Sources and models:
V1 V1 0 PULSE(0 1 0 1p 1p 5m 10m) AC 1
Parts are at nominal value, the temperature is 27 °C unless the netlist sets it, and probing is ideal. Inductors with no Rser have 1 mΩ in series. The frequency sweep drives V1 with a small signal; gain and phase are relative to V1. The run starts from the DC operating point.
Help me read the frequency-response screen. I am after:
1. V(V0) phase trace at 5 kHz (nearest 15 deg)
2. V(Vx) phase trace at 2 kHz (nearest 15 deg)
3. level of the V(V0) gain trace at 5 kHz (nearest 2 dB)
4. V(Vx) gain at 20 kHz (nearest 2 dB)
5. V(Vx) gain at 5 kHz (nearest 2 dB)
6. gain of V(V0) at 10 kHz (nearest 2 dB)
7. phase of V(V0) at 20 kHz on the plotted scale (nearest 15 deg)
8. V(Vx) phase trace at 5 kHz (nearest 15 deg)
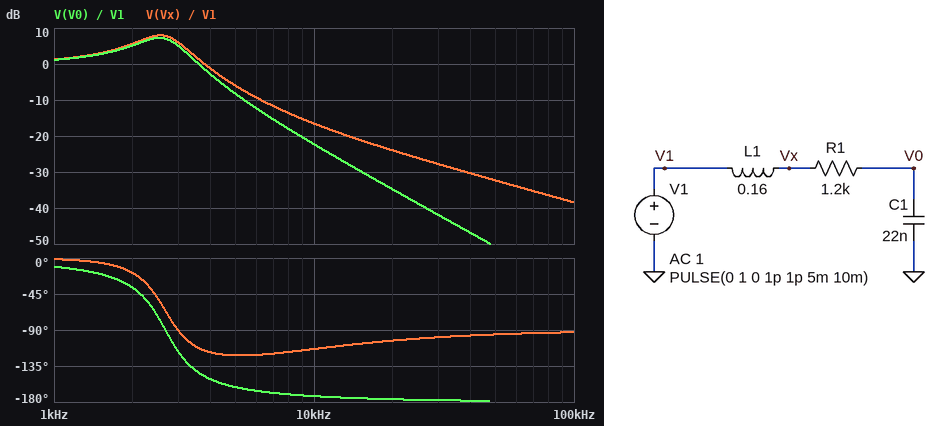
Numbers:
-165 deg
-15 deg
-8 dB
-24 dB
-6 dB
-22 dB
-180 deg
-120 deg
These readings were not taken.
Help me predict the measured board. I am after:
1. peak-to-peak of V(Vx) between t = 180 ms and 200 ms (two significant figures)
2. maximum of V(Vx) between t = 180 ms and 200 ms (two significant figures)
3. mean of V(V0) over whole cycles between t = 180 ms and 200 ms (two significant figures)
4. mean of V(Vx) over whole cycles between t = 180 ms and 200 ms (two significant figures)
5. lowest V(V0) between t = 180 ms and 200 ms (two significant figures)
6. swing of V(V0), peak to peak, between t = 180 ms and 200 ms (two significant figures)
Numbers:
2.1 V
1.5 V
500 mV
500 mV
-490 mV
2.0 V
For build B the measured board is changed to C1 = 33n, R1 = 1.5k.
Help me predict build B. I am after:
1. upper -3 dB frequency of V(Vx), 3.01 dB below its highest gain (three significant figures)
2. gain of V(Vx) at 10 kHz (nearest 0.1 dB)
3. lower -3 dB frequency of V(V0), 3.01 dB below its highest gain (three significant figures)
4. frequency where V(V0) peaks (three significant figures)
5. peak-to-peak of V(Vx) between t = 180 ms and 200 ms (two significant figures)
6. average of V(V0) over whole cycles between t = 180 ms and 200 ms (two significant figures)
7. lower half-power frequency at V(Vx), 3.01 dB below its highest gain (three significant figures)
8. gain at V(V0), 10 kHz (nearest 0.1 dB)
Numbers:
2.73 kHz
-15.8 dB
782 Hz
1.92 kHz
1.8 V
500 mV
1.11 kHz
-26.1 dB
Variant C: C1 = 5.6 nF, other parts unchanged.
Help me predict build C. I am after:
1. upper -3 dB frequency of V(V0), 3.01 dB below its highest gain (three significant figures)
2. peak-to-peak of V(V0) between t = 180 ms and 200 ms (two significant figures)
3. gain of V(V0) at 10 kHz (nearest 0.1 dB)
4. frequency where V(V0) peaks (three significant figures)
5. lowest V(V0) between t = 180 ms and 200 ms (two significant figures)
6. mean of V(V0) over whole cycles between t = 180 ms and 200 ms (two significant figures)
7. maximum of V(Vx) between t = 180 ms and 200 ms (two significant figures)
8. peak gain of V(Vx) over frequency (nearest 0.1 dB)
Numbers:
5.82 kHz
2.4 V
-8.2 dB
5.25 kHz
-700 mV
500 mV
1.7 V
13.2 dB
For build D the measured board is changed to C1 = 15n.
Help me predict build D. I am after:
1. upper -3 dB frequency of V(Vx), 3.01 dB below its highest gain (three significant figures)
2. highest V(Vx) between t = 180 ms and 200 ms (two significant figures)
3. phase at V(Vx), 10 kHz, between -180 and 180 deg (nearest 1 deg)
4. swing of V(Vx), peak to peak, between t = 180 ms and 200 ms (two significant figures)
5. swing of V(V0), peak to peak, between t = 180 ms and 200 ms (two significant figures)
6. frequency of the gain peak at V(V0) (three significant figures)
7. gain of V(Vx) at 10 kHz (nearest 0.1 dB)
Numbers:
3.72 kHz
1.6 V
-124 deg
2.2 V
2.1 V
3.14 kHz
-15.1 dB
